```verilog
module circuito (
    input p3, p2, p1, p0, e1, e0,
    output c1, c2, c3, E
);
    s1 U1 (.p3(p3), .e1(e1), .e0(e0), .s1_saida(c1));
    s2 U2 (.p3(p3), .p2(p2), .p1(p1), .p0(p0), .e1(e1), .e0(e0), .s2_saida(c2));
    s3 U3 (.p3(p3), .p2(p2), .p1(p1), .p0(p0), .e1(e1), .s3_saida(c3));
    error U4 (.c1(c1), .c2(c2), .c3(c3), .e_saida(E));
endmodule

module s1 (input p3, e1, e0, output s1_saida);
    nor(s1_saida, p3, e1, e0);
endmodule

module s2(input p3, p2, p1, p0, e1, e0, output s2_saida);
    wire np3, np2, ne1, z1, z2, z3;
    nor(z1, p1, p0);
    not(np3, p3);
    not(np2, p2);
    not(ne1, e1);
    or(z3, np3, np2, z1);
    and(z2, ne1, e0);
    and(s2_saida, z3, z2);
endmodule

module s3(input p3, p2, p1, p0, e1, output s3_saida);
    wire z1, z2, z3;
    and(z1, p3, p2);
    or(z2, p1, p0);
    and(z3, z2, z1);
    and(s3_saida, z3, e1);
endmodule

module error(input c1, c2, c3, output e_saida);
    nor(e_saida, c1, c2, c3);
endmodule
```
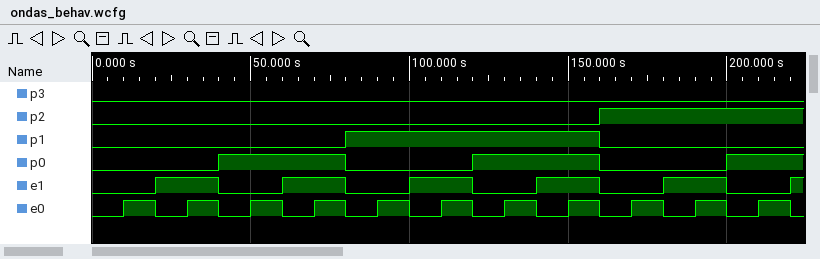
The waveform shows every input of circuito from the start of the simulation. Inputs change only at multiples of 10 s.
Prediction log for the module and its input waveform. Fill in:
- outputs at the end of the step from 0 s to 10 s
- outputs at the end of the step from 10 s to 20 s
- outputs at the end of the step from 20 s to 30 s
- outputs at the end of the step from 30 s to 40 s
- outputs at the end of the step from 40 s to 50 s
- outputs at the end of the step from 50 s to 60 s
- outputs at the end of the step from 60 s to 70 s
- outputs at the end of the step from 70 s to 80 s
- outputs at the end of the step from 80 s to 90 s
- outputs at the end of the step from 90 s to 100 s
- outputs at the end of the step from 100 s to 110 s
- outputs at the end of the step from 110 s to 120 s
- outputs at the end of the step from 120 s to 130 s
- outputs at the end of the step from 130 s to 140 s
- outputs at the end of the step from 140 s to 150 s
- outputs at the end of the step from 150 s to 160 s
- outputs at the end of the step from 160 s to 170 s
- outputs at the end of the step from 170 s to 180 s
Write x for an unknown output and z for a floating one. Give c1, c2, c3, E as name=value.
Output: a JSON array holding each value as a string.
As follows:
["c1=1, c2=0, c3=0, E=0", "c1=0, c2=1, c3=0, E=0", "c1=0, c2=0, c3=0, E=1", "c1=0, c2=0, c3=0, E=1", "c1=1, c2=0, c3=0, E=0", "c1=0, c2=1, c3=0, E=0", "c1=0, c2=0, c3=0, E=1", "c1=0, c2=0, c3=0, E=1", "c1=1, c2=0, c3=0, E=0", "c1=0, c2=1, c3=0, E=0", "c1=0, c2=0, c3=0, E=1", "c1=0, c2=0, c3=0, E=1", "c1=1, c2=0, c3=0, E=0", "c1=0, c2=1, c3=0, E=0", "c1=0, c2=0, c3=0, E=1", "c1=0, c2=0, c3=0, E=1", "c1=1, c2=0, c3=0, E=0", "c1=0, c2=1, c3=0, E=0"]
